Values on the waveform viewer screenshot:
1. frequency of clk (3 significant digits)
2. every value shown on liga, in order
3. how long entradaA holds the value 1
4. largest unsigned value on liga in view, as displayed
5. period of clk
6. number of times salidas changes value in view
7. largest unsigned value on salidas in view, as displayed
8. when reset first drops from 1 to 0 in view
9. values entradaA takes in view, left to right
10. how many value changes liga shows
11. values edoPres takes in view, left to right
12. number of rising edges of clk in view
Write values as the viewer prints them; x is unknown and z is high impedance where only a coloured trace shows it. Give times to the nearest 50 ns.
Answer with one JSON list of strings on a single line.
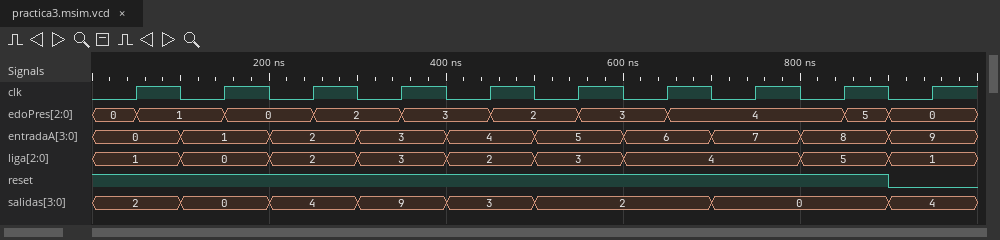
["10.0 MHz", "1, 0, 2, 3, 2, 3, 4, 5, 1", "100 ns", "5", "100 ns", "7", "9", "900 ns", "0, 1, 2, 3, 4, 5, 6, 7, 8, 9", "8", "0, 1, 0, 2, 3, 2, 3, 4, 5, 0", "10"]
